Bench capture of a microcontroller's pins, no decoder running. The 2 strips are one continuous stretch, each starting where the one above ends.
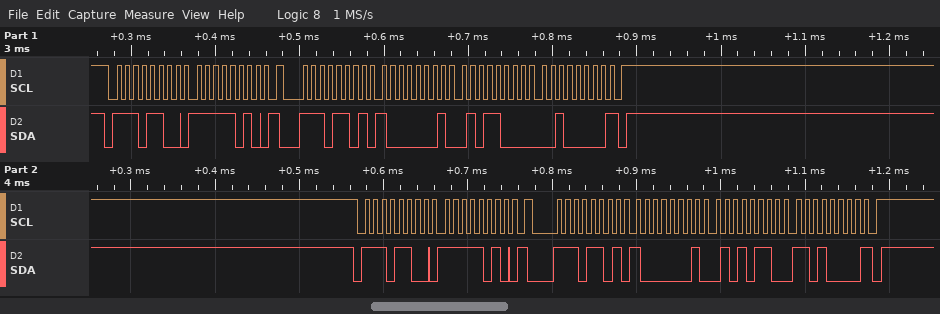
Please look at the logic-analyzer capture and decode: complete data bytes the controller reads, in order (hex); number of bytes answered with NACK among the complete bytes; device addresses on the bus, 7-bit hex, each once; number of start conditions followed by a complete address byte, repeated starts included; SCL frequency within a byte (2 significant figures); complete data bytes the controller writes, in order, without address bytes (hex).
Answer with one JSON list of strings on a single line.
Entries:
["81 58 20 81 56 D0", "2", "0x76", "4", "100 kHz", "FA FA"]
